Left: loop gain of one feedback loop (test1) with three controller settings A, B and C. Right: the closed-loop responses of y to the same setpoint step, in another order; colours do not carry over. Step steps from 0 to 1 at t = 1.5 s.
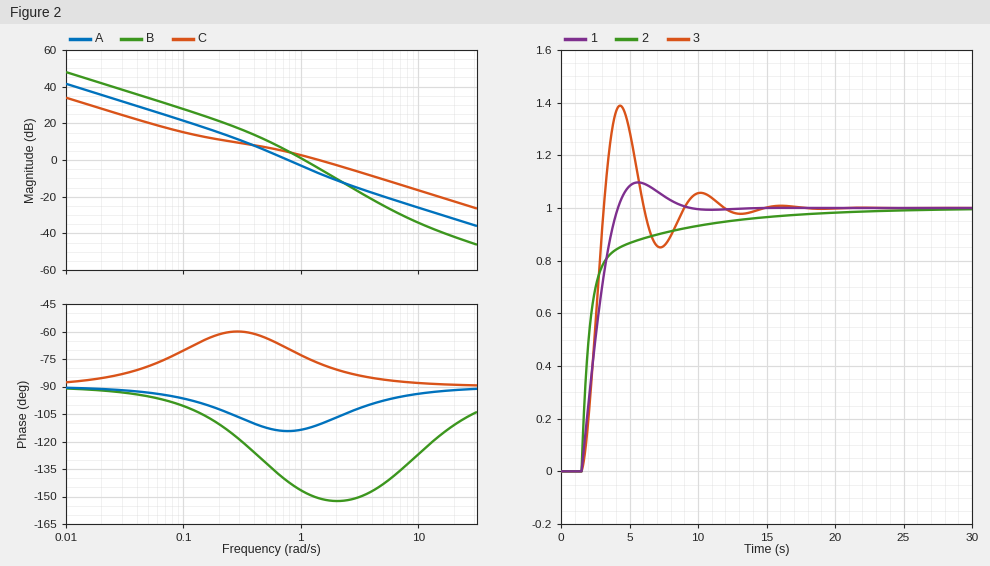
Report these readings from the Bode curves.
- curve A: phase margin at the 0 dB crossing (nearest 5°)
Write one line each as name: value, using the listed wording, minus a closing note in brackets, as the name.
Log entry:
curve A: phase margin at the 0 dB crossing: 65°
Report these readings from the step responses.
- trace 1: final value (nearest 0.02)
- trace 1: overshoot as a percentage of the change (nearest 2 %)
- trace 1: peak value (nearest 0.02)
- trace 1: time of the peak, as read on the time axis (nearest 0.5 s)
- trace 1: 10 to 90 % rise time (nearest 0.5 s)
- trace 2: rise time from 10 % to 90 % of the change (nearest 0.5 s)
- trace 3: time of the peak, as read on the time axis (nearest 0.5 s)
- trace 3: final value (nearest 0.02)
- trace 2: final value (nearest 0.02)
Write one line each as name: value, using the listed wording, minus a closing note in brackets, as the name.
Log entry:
trace 1: final value: 1.00
trace 1: overshoot as a percentage of the change: 10 %
trace 1: peak value: 1.10
trace 1: time of the peak, as read on the time axis: 5.5 s
trace 1: 10 to 90 % rise time: 2.0 s
trace 2: rise time from 10 % to 90 % of the change: 5.5 s
trace 3: time of the peak, as read on the time axis: 4.5 s
trace 3: final value: 1.00
trace 2: final value: 1.00
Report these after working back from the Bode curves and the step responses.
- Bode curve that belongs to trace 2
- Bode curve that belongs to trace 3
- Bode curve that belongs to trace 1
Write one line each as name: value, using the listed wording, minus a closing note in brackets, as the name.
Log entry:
Bode curve that belongs to trace 2: C
Bode curve that belongs to trace 3: B
Bode curve that belongs to trace 1: A
